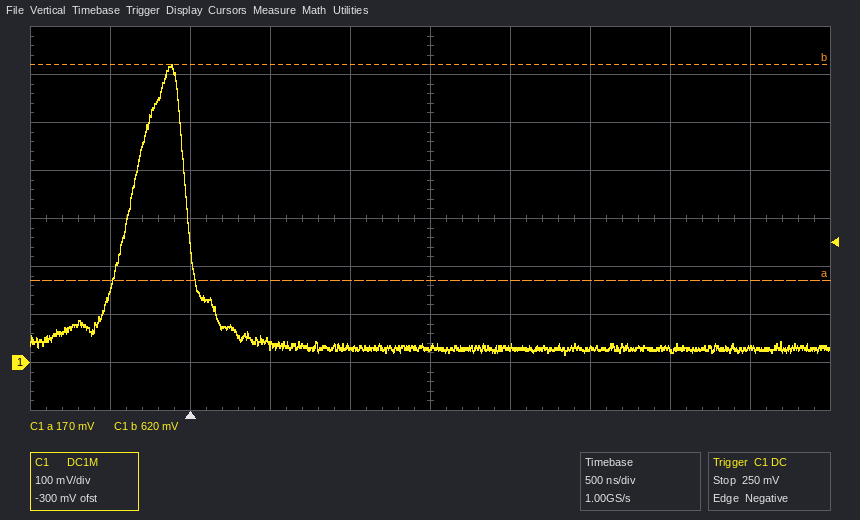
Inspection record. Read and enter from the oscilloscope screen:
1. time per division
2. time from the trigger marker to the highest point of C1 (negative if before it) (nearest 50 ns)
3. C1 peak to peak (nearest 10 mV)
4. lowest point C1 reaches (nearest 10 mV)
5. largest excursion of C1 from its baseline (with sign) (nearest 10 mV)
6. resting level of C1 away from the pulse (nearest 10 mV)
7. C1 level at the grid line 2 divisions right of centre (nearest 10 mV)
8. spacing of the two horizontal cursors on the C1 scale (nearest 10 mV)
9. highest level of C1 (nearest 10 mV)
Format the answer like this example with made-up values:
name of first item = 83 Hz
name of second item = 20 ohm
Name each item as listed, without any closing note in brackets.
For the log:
time per division = 500 ns
time from the trigger marker to the highest point of C1 (negative if before it) = -100 ns
C1 peak to peak = 600 mV
lowest point C1 reaches = 20 mV
largest excursion of C1 from its baseline (with sign) = +590 mV
resting level of C1 away from the pulse = 30 mV
C1 level at the grid line 2 divisions right of centre = 30 mV
spacing of the two horizontal cursors on the C1 scale = 450 mV
highest level of C1 = 620 mV
